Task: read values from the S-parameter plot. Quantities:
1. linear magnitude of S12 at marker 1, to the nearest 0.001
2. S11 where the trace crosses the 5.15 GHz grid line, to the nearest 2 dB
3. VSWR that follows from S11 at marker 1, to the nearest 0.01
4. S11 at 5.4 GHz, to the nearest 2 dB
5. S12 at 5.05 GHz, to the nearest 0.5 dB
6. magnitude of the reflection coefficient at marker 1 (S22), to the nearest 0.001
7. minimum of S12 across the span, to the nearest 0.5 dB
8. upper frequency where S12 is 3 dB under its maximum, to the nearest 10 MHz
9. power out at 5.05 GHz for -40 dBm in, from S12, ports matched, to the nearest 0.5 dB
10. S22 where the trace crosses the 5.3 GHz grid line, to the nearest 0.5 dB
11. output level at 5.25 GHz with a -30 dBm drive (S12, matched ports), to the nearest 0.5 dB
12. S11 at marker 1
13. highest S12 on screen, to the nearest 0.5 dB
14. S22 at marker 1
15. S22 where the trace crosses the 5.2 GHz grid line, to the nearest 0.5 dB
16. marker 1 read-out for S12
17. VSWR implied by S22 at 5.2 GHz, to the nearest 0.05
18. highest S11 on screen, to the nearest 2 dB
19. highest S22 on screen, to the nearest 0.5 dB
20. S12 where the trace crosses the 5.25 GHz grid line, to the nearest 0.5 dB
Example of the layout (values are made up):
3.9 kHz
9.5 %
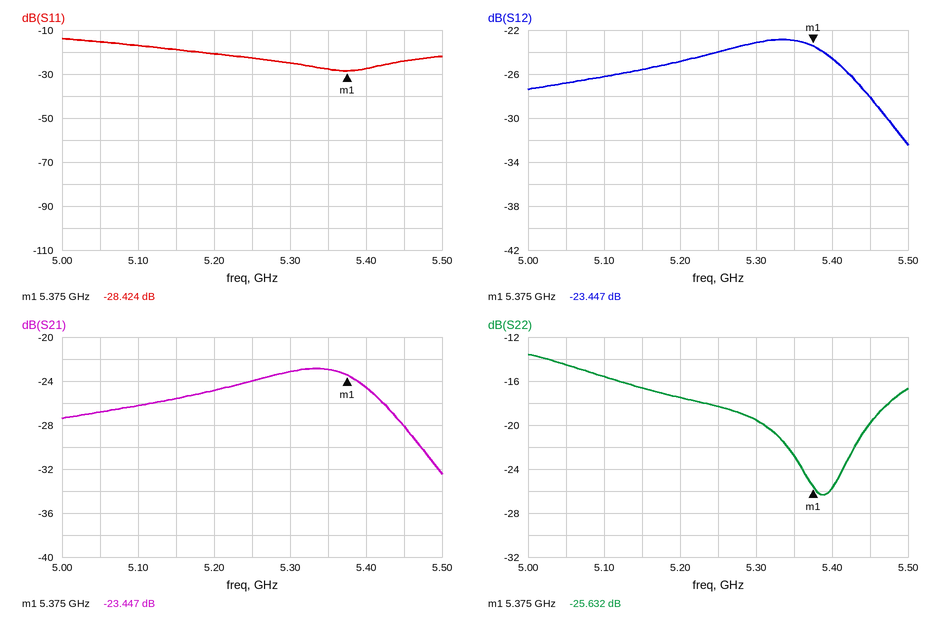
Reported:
0.067
-18 dB
1.08
-28 dB
-27.0 dB
0.052
-32.5 dB
5.42 GHz
-67.0 dBm
-19.5 dB
-54.0 dBm
-28.424 dB
-23.0 dB
-25.632 dB
-17.5 dB
-23.447 dB
1.30
-14 dB
-13.5 dB
-24.0 dB
